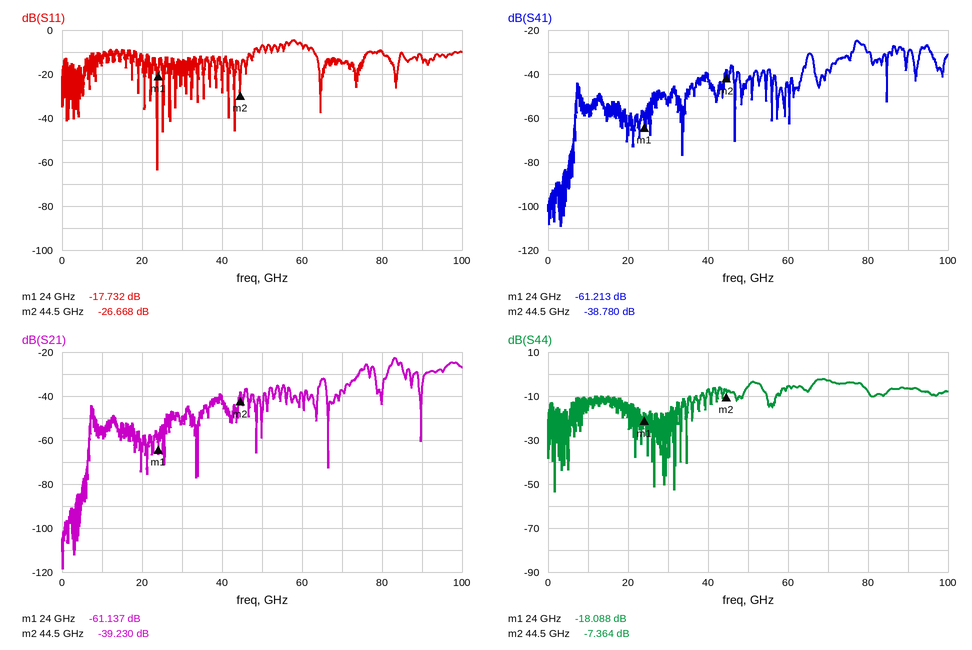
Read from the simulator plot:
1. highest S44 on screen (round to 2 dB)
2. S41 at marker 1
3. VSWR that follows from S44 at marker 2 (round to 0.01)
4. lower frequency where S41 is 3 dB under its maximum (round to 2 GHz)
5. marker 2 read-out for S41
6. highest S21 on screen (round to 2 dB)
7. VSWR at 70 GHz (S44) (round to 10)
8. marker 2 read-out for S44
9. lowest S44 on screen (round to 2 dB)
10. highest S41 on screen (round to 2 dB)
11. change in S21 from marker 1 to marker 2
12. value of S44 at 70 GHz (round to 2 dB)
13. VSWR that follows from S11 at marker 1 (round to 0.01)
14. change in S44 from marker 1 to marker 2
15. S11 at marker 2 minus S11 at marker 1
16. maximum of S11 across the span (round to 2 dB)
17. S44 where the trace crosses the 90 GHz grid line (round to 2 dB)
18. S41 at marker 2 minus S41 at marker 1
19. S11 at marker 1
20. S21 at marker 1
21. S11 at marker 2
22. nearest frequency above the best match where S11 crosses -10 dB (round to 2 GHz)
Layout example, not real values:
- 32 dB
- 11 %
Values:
- -2 dB
- -61.213 dB
- 2.50
- 76 GHz
- -38.780 dB
- -22 dB
- 10
- -7.364 dB
- -54 dB
- -24 dB
- 21.907 dB
- -2 dB
- 1.30
- 10.724 dB
- -8.936 dB
- -4 dB
- -6 dB
- 22.433 dB
- -17.732 dB
- -61.137 dB
- -26.668 dB
- 48 GHz
